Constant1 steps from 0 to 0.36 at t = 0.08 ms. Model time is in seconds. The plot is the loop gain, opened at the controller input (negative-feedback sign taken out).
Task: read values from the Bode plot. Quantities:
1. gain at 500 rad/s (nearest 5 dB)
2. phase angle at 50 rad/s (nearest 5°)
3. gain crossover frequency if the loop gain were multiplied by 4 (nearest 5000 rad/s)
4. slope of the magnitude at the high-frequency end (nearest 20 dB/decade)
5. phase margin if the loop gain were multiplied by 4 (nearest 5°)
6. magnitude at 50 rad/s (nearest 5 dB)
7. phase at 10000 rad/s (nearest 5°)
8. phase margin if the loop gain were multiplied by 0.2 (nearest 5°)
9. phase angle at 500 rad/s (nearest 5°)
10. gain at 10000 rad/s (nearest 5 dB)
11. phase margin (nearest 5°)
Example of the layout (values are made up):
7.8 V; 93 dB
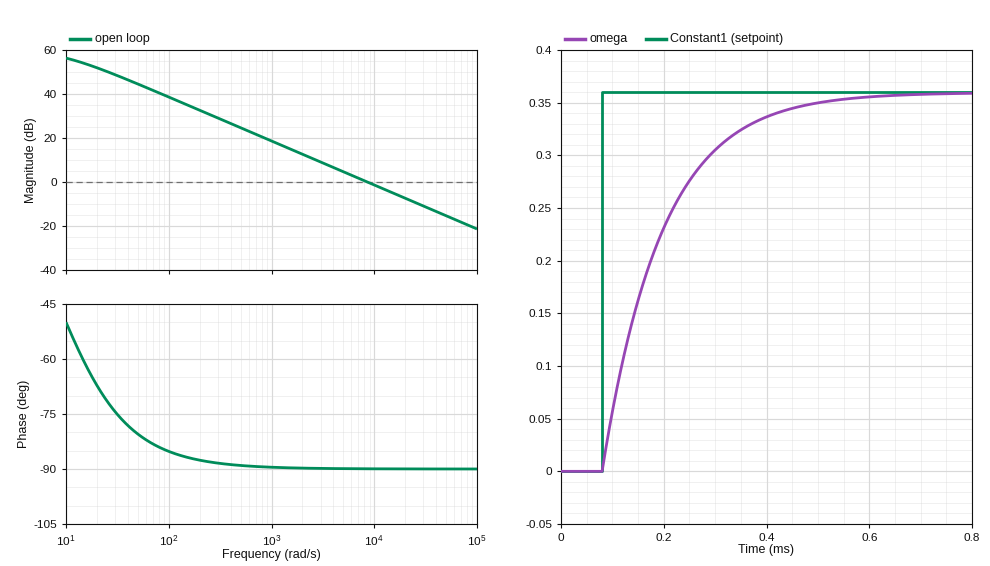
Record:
25 dB; -80°; 35000 rad/s; -20 dB/decade; 90°; 45 dB; -90°; 90°; -90°; 0 dB; 90°
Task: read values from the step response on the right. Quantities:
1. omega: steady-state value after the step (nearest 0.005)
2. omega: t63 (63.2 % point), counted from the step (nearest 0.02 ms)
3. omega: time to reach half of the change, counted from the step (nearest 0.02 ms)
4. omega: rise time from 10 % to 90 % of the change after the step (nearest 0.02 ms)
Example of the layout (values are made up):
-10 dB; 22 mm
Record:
0.360; 0.12 ms; 0.08 ms; 0.26 ms
